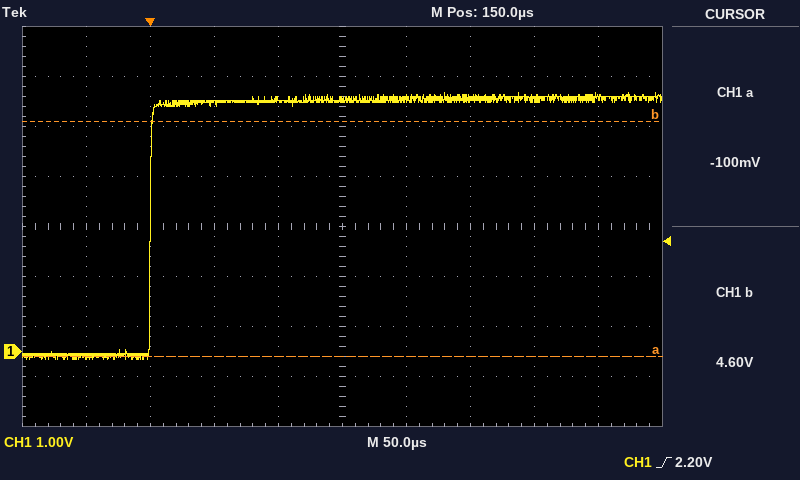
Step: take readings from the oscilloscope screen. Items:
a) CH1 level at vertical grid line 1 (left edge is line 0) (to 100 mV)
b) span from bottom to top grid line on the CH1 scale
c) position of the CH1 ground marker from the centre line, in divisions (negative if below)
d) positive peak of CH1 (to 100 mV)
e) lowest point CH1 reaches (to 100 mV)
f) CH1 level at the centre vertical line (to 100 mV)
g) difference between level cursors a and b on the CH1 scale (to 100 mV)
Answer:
-100 mV
8 V
-2.5 div
5.2 V
-200 mV
5.0 V
4.7 V
